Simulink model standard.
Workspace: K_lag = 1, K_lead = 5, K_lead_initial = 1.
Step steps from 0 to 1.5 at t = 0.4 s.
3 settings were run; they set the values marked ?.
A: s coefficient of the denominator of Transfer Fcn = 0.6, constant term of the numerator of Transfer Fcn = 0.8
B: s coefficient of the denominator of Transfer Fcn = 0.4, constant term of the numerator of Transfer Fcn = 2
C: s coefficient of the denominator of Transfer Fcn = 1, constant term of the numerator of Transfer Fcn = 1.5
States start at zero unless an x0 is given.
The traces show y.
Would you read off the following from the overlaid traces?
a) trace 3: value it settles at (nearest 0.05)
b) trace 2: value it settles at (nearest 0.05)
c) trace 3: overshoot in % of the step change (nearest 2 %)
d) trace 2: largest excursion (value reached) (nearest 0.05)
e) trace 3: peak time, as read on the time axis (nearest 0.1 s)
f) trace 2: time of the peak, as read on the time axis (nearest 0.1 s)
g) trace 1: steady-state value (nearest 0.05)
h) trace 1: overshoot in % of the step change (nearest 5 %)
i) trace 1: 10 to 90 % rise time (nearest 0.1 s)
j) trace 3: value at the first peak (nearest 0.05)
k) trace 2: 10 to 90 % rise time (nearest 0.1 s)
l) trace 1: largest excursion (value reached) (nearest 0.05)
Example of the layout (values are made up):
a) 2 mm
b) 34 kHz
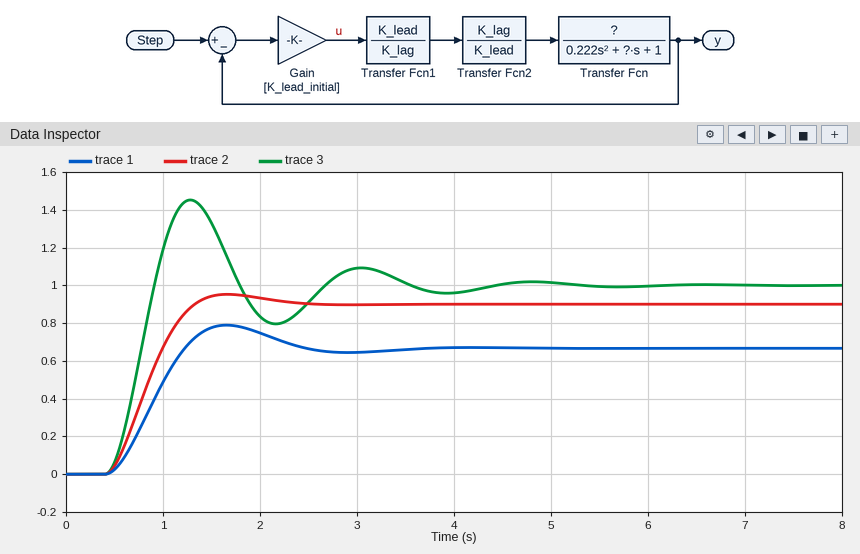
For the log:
a) 1.00
b) 0.90
c) 46 %
d) 0.95
e) 1.3 s
f) 1.7 s
g) 0.65
h) 20 %
i) 0.6 s
j) 1.45
k) 0.6 s
l) 0.80
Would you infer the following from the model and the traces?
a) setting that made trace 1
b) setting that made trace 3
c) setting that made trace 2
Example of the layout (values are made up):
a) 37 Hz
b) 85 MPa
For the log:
a) A
b) B
c) C
